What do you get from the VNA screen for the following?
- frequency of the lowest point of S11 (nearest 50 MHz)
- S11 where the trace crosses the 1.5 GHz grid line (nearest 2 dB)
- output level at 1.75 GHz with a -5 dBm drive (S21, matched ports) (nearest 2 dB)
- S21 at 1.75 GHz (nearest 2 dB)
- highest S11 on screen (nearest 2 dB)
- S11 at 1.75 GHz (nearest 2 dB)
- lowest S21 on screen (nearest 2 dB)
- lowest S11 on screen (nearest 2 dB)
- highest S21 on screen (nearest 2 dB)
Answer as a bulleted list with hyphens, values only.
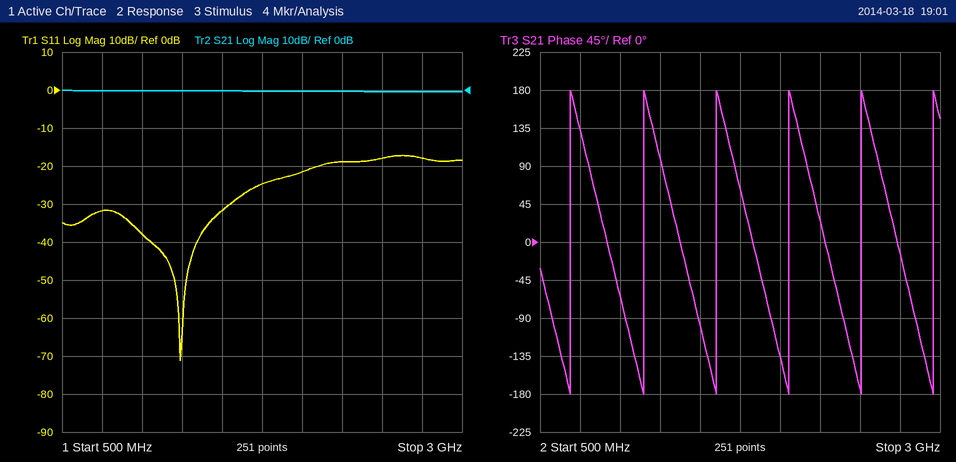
- 1.25 GHz
- -32 dB
- -6 dBm
- 0 dB
- -18 dB
- -24 dB
- 0 dB
- -72 dB
- 0 dB
